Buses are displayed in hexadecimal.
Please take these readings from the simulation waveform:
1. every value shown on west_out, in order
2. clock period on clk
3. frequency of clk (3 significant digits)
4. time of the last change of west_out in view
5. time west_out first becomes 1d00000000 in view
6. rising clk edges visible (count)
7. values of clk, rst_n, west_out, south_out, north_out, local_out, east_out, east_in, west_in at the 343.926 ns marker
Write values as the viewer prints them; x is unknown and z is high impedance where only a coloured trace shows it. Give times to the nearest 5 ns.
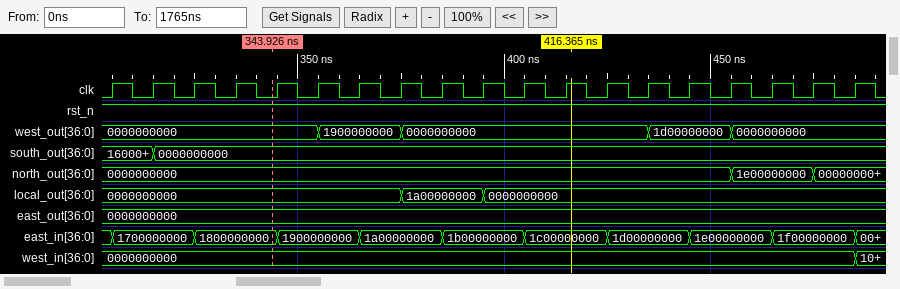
0000000000, 1900000000, 0000000000, 1d00000000, 0000000000
10 ns
100 MHz
455 ns
435 ns
19
clk=0, rst_n=1, west_out=0000000000, south_out=0000000000, north_out=0000000000, local_out=0000000000, east_out=0000000000, east_in=1800000000, west_in=0000000000
